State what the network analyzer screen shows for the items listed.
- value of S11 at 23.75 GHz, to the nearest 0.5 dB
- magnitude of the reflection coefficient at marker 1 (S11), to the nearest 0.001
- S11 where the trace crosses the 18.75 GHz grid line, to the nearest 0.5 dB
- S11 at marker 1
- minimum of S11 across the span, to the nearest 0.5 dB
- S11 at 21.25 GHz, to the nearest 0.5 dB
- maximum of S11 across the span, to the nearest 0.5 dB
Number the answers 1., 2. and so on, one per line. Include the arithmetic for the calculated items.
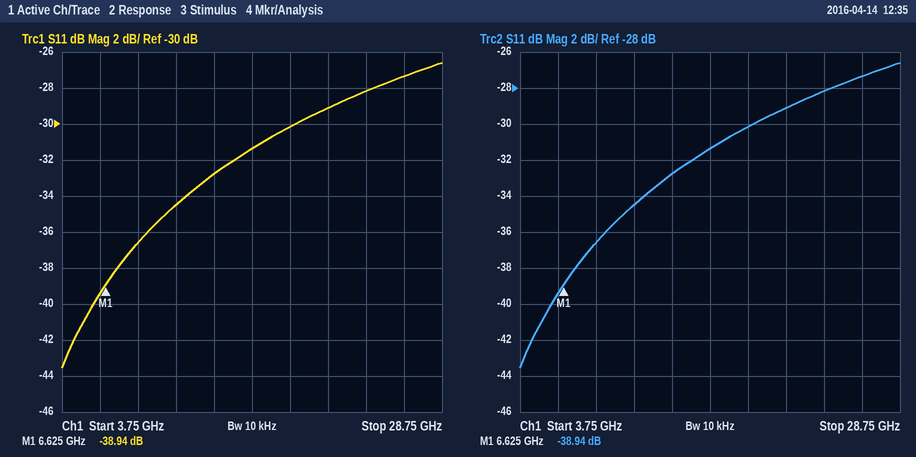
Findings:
1. -28.0 dB
2. 10^(-38.94/20) ≈ 0.011
3. -30.0 dB
4. -38.94 dB
5. -43.5 dB
6. -29.0 dB
7. -26.5 dB
